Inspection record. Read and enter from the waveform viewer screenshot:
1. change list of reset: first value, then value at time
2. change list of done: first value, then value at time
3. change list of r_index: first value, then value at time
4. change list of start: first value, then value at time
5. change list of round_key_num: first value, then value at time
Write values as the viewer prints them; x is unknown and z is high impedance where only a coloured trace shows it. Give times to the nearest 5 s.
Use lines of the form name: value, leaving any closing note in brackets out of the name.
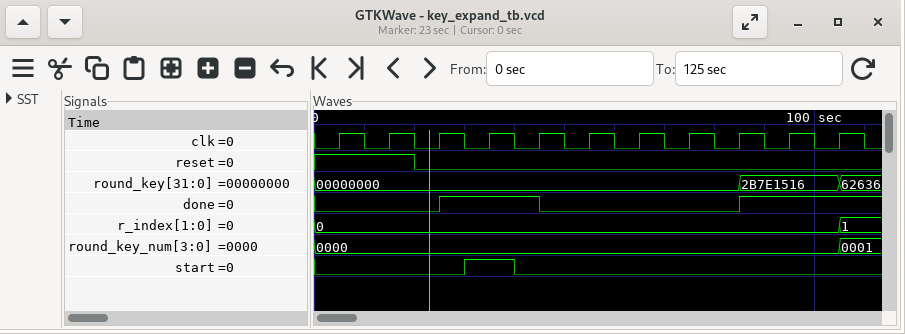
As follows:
change list of reset: first value, then value at time: 1, 0 at 20 s
change list of done: first value, then value at time: 0, 1 at 25 s, 0 at 45 s, 1 at 85 s
change list of r_index: first value, then value at time: 0, 1 at 105 s
change list of start: first value, then value at time: 0, 1 at 30 s, 0 at 40 s
change list of round_key_num: first value, then value at time: 0000, 0001 at 105 s
